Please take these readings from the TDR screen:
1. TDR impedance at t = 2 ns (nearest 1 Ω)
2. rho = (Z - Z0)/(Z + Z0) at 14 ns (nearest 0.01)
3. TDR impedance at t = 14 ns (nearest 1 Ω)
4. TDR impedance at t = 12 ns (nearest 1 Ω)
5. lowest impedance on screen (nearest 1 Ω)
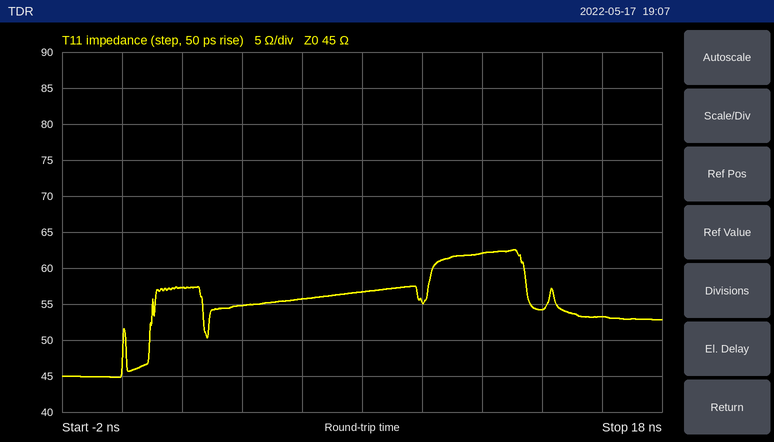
57 Ω
+0.09
54 Ω
62 Ω
45 Ω
